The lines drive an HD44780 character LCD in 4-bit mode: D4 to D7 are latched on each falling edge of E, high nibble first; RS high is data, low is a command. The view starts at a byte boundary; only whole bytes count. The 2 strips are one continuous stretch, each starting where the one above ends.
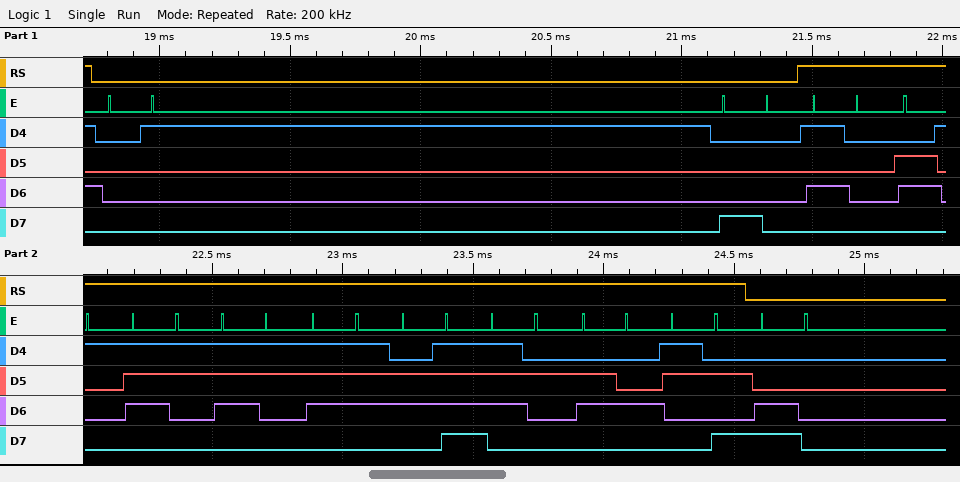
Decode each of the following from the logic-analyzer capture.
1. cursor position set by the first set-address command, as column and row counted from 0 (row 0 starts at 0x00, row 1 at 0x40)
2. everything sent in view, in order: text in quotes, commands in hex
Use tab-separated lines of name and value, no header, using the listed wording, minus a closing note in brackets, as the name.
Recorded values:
cursor position set by the first set-address command, as column and row counted from 0	column 0, row 0
everything sent in view, in order: text in quotes, commands in hex	0x01 0x80 "Password:" 0xC0
